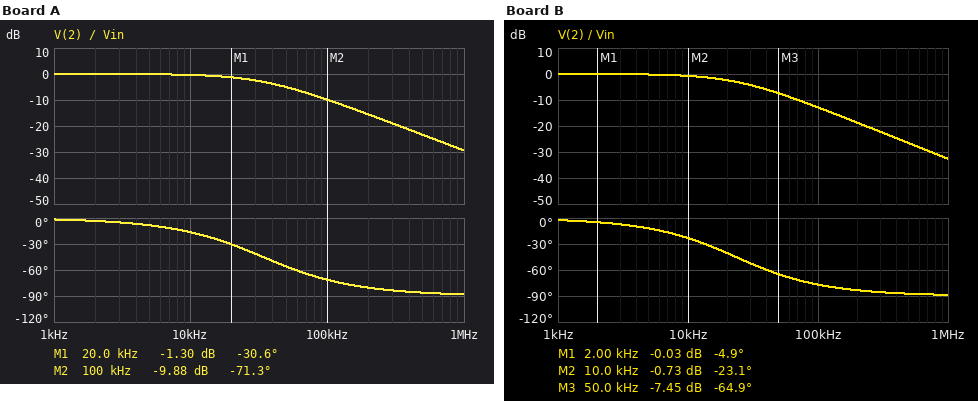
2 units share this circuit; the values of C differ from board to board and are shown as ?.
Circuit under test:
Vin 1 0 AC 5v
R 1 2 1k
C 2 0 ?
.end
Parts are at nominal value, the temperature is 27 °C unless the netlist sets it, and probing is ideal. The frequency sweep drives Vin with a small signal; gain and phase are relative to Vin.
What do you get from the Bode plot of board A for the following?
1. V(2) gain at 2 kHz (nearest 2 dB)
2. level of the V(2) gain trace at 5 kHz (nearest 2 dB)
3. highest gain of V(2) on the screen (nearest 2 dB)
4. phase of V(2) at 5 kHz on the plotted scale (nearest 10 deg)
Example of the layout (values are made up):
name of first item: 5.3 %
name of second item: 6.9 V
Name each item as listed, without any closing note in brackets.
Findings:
V(2) gain at 2 kHz: 0 dB
level of the V(2) gain trace at 5 kHz: 0 dB
highest gain of V(2) on the screen: 0 dB
phase of V(2) at 5 kHz on the plotted scale: -10 deg
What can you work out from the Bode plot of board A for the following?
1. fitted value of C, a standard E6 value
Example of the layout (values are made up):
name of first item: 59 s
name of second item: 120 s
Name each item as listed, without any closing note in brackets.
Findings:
fitted value of C, a standard E6 value: 4.7 nF
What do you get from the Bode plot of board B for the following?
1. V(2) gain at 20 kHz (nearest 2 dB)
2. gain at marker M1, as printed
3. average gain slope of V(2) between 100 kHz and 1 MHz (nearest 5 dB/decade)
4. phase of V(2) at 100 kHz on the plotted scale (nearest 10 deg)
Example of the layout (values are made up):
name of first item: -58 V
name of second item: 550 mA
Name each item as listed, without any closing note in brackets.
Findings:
V(2) gain at 20 kHz: -2 dB
gain at marker M1, as printed: -0.03 dB
average gain slope of V(2) between 100 kHz and 1 MHz: -20 dB/decade
phase of V(2) at 100 kHz on the plotted scale: -80 deg
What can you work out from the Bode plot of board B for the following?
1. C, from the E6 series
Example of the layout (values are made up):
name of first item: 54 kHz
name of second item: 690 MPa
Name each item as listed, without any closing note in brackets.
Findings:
C, from the E6 series: 6.8 nF
